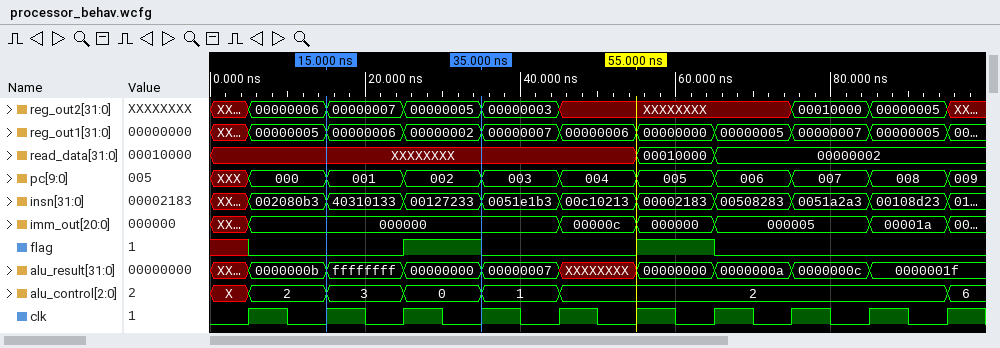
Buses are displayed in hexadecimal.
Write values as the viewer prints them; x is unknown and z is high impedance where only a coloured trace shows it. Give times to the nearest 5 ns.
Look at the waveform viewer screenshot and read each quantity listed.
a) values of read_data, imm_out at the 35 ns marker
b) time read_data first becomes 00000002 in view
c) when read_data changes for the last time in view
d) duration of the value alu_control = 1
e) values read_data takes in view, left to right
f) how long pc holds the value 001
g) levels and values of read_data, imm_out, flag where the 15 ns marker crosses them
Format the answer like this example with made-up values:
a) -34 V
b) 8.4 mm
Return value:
a) read_data=XXXXXXXX, imm_out=000000
b) 65 ns
c) 65 ns
d) 10 ns
e) XXXXXXXX, 00010000, 00000002
f) 10 ns
g) read_data=XXXXXXXX, imm_out=000000, flag=0
